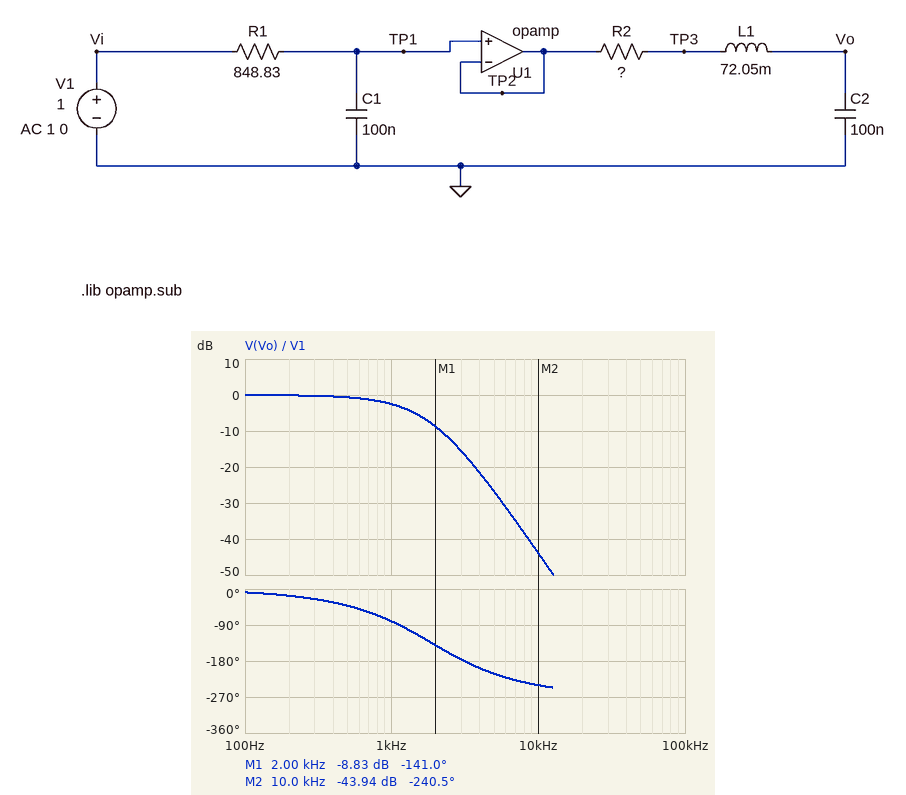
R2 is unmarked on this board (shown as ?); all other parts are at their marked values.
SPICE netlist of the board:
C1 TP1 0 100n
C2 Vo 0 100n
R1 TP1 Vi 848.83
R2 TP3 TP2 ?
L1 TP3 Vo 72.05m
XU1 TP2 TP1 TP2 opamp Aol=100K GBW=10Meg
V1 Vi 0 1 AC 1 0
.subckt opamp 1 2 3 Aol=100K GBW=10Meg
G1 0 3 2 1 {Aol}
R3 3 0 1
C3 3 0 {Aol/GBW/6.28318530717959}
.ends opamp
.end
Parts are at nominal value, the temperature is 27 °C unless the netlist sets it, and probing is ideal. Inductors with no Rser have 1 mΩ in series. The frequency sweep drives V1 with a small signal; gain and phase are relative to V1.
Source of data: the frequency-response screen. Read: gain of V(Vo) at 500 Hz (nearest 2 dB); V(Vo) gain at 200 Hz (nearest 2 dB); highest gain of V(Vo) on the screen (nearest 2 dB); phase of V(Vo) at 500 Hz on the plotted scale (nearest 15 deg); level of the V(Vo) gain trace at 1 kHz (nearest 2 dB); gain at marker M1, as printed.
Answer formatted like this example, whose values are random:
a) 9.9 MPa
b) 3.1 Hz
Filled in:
a) 0 dB
b) 0 dB
c) 0 dB
d) -45 deg
e) -2 dB
f) -8.83 dB
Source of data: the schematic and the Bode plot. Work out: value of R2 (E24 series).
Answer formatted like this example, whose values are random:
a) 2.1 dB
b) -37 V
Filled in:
a) 1.5 kΩ
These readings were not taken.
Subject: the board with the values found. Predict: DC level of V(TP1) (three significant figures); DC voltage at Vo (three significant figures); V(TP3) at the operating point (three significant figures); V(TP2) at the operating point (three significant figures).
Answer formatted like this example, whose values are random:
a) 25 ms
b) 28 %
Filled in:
a) 1.00 V
b) 1.00 V
c) 1.00 V
d) 1.00 V
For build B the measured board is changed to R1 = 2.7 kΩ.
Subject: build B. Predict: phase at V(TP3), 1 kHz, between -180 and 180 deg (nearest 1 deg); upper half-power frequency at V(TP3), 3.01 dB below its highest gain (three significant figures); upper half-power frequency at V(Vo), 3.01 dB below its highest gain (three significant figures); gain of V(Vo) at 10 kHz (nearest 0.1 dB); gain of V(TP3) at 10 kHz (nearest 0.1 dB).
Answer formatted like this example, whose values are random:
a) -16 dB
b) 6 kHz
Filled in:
a) -112 deg
b) 470 Hz
c) 534 Hz
d) -53.9 dB
e) -25.1 dB
